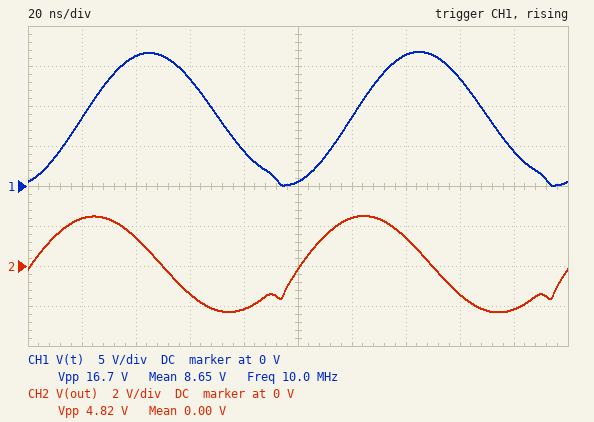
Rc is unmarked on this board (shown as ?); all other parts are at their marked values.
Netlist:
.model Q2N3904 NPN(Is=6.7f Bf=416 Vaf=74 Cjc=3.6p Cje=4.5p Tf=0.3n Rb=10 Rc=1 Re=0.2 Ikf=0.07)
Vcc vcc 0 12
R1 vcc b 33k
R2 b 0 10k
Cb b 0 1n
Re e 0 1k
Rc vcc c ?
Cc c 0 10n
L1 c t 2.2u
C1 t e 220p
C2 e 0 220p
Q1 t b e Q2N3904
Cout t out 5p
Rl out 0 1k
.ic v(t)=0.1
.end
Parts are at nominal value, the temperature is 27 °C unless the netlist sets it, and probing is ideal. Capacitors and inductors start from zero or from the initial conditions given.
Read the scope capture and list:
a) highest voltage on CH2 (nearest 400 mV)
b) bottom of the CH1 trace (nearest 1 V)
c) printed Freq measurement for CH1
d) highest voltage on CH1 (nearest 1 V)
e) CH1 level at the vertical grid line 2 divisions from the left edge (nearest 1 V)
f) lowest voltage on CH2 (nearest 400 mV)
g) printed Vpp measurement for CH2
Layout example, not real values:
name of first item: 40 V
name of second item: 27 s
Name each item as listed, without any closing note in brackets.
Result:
highest voltage on CH2: 2.4 V
bottom of the CH1 trace: 0 V
printed Freq measurement for CH1: 10.0 MHz
highest voltage on CH1: 17 V
CH1 level at the vertical grid line 2 divisions from the left edge: 16 V
lowest voltage on CH2: -2.4 V
printed Vpp measurement for CH2: 4.82 V
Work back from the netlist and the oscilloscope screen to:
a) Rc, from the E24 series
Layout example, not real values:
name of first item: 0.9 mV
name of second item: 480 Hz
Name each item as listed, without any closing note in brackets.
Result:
Rc, from the E24 series: 390 Ω
